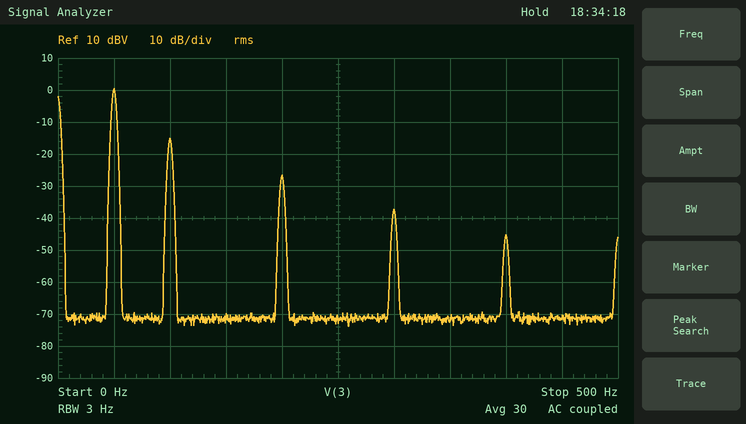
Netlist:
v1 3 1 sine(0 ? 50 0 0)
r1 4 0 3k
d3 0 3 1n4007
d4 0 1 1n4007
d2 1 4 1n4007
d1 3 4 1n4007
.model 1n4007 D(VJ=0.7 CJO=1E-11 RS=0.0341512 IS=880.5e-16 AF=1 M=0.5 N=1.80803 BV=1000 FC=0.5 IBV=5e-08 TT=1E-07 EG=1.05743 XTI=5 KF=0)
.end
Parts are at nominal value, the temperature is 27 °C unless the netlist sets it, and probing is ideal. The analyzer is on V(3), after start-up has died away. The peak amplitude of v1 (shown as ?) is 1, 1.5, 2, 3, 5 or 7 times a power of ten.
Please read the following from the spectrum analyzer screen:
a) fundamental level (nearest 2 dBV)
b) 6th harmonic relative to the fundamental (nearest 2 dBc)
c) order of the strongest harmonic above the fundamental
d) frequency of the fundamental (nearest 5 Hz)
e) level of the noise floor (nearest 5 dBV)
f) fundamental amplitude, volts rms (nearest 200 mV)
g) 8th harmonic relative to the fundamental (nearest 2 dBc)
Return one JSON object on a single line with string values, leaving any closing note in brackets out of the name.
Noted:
{"fundamental level": "0 dBV", "6th harmonic relative to the fundamental": "-38 dBc", "order of the strongest harmonic above the fundamental": "2", "frequency of the fundamental": "50 Hz", "level of the noise floor": "-70 dBV", "fundamental amplitude, volts rms": "1.0 V", "8th harmonic relative to the fundamental": "-46 dBc"}
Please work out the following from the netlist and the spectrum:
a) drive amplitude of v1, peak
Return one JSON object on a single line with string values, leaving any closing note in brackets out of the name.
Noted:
{"drive amplitude of v1, peak": "3 V"}
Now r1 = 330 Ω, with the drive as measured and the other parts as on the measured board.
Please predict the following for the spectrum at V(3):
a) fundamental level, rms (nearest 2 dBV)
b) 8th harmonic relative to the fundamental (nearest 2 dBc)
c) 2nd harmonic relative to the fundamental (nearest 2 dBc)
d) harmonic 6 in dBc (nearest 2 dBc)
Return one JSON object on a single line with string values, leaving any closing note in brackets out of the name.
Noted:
{"fundamental level, rms": "0 dBV", "8th harmonic relative to the fundamental": "-42 dBc", "2nd harmonic relative to the fundamental": "-18 dBc", "harmonic 6 in dBc": "-48 dBc"}
